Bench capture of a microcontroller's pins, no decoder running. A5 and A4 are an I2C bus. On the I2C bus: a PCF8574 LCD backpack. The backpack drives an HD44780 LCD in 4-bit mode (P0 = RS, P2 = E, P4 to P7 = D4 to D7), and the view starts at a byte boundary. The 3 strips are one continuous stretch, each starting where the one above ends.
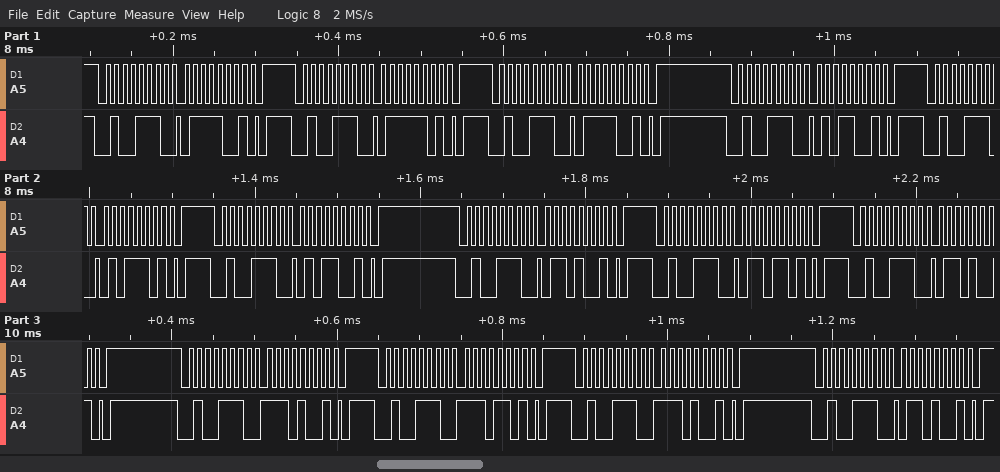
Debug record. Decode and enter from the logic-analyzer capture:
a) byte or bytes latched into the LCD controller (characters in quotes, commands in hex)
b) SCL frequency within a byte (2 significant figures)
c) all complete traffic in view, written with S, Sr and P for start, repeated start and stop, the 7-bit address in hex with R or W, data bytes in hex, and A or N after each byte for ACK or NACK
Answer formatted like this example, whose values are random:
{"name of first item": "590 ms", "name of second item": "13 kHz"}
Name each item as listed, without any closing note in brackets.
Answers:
{"byte or bytes latched into the LCD controller": "'u' 'n'", "SCL frequency within a byte": "100 kHz", "all complete traffic in view, written with S, Sr and P for start, repeated start and stop, the 7-bit address in hex with R or W, data bytes in hex, and A or N after each byte for ACK or NACK": "S 27W A 79 A P S 27W A 7D A P S 27W A 79 A P S 27W A 59 A P S 27W A 5D A P S 27W A 59 A P S 27W A 69 A P S 27W A 6D A P S 27W A 69 A P S 27W A E9 A P S 27W A ED A P S 27W A E9 A P S 27W A 69 A P"}
